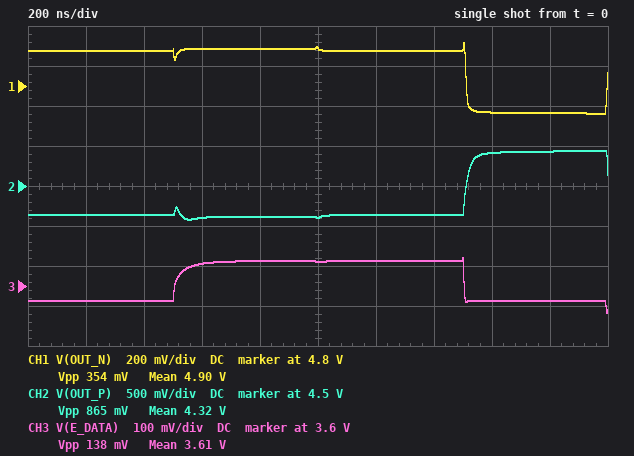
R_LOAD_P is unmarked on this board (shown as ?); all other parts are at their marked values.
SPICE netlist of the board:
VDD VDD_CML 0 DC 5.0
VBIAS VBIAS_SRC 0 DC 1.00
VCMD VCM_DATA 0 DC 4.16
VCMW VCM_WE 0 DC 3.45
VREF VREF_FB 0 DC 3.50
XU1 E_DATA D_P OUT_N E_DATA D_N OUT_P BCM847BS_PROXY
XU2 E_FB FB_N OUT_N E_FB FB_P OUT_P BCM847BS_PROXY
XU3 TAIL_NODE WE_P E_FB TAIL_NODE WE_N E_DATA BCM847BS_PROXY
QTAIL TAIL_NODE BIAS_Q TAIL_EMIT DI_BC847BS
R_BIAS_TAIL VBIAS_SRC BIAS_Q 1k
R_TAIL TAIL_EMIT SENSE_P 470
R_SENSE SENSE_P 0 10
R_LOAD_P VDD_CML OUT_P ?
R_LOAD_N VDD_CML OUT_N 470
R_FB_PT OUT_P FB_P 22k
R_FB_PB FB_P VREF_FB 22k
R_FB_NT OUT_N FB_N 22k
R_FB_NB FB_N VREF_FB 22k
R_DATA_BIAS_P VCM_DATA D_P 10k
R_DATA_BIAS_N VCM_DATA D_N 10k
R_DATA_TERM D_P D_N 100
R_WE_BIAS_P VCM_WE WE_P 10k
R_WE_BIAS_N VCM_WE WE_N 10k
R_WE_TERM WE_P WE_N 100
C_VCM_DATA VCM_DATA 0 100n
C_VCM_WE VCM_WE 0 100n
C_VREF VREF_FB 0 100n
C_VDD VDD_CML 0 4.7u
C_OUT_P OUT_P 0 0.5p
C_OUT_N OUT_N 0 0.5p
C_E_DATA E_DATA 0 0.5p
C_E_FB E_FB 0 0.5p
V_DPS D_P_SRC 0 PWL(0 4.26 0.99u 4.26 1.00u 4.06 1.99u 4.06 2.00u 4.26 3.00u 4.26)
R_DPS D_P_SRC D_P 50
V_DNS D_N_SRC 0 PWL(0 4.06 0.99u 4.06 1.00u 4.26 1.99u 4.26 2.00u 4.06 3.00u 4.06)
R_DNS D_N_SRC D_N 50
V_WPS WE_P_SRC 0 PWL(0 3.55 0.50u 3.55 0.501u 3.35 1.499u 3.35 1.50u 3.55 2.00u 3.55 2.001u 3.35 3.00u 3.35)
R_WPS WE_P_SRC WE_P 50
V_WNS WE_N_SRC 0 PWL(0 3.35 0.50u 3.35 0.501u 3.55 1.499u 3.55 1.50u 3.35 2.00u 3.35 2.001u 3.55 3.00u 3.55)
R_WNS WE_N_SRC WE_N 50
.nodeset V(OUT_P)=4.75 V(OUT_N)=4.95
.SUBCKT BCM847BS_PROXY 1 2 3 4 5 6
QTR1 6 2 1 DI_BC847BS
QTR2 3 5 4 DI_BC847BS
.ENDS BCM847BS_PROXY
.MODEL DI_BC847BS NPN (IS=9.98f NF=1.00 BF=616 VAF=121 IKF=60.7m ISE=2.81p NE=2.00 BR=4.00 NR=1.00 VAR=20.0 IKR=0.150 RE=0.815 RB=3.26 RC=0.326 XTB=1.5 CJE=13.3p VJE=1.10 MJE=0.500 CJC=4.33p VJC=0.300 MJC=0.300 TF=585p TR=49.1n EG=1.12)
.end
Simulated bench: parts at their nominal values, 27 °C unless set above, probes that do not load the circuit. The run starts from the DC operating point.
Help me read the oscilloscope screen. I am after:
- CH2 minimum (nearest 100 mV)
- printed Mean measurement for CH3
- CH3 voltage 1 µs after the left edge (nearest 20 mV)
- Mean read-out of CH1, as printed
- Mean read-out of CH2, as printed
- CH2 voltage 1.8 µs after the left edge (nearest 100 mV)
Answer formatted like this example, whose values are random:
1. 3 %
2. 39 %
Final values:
1. 4.1 V
2. 3.61 V
3. 3.66 V
4. 4.90 V
5. 4.32 V
6. 4.9 V
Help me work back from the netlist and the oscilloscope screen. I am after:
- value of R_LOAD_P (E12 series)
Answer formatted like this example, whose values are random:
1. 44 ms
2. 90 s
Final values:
1. 1.2 kΩ
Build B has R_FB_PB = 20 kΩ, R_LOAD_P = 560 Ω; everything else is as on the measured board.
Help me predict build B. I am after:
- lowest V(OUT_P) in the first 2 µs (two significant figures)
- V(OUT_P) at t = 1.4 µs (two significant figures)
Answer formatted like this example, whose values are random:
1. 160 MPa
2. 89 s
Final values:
1. 4.5 V
2. 4.6 V
